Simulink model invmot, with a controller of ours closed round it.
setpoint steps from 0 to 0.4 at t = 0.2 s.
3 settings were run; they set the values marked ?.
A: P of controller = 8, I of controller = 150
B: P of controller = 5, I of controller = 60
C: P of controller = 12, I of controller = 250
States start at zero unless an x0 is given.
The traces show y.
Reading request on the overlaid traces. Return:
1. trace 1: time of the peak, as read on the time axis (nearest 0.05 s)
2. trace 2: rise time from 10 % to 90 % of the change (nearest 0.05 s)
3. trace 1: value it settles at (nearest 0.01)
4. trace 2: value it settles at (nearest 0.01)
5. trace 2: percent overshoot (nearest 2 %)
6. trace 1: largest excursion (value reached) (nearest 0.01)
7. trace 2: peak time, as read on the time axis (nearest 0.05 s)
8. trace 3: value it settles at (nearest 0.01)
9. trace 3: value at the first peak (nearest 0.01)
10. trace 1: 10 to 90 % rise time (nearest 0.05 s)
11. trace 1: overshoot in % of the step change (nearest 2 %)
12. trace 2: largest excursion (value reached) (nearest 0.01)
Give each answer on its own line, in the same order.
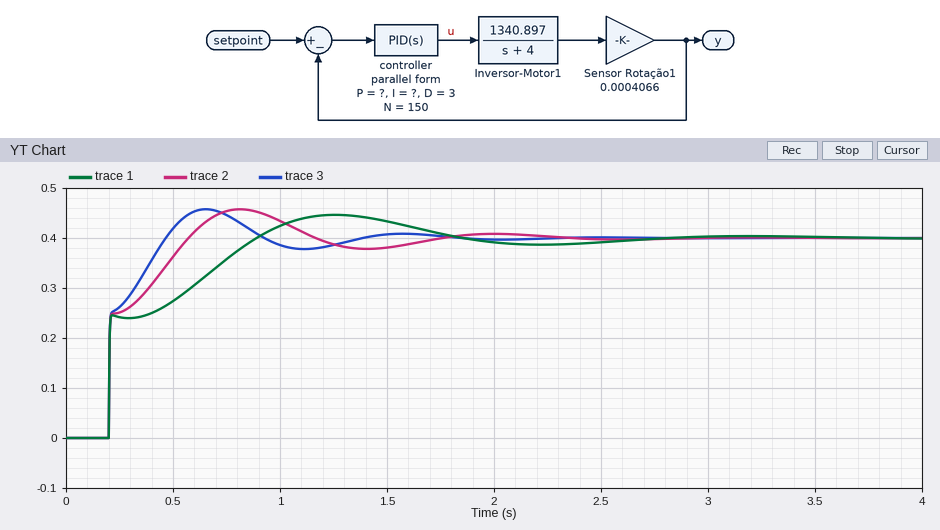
1.25 s
0.30 s
0.40
0.40
14 %
0.45
0.80 s
0.40
0.46
0.55 s
12 %
0.46
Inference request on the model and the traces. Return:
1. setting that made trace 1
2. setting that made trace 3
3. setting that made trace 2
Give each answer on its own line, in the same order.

B
C
A
